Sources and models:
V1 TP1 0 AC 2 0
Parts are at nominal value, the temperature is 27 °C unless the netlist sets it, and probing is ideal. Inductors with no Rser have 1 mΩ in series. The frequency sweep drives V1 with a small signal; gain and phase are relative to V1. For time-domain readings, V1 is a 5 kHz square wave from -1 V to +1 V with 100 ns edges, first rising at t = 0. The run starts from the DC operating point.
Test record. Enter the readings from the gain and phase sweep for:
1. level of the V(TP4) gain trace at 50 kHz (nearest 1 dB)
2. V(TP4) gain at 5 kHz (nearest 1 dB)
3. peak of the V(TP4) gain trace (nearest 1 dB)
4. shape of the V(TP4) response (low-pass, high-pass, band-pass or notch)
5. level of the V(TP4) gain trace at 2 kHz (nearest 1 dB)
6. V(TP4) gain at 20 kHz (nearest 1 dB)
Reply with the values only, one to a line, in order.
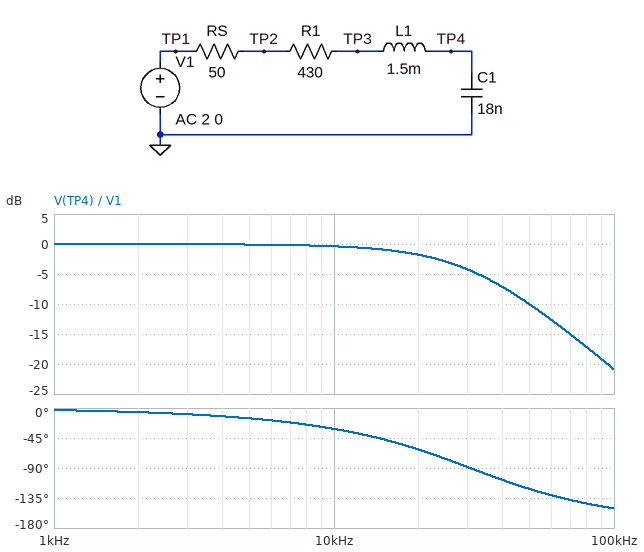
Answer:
-10 dB
0 dB
0 dB
low-pass
0 dB
-2 dB
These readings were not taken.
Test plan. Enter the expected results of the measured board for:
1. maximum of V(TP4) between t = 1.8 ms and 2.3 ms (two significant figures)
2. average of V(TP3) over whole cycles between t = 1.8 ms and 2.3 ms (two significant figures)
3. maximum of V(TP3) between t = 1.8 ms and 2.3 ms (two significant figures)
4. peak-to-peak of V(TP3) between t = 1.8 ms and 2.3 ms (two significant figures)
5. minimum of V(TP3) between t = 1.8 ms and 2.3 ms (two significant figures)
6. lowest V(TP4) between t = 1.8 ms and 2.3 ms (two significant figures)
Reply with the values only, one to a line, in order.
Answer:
1.0 V
160 mV
1.0 V
2.0 V
-1.0 V
-1.0 V
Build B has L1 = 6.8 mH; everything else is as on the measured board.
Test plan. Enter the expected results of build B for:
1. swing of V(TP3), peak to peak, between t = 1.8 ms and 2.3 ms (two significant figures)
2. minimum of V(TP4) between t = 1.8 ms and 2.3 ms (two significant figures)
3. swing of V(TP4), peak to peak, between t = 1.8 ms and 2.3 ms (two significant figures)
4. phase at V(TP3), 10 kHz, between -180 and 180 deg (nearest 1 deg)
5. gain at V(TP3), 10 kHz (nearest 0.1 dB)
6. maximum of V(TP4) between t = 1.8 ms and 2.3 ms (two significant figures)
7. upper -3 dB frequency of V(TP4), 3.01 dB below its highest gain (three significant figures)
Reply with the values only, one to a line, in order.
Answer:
2.5 V
-1.5 V
3.1 V
-46 deg
-3.2 dB
1.5 V
17.1 kHz
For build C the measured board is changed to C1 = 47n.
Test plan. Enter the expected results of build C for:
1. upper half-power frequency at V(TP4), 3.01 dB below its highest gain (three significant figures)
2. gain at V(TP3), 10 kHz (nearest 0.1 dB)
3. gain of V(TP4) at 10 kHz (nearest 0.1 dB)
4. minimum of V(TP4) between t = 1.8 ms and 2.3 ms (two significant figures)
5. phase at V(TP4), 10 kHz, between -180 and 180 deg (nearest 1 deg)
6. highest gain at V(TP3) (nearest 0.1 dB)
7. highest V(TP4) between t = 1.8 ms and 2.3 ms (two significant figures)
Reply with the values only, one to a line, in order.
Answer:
8.15 kHz
-6.9 dB
-4.0 dB
-990 mV
-63 deg
0 dB
990 mV
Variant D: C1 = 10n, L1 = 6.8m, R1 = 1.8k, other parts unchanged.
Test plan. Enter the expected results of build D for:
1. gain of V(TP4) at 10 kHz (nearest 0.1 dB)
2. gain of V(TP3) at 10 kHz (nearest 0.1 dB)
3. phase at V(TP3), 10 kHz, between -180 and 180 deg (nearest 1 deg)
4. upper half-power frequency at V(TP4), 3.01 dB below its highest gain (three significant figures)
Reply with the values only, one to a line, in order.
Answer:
-2.8 dB
-5.5 dB
-58 deg
10.6 kHz
